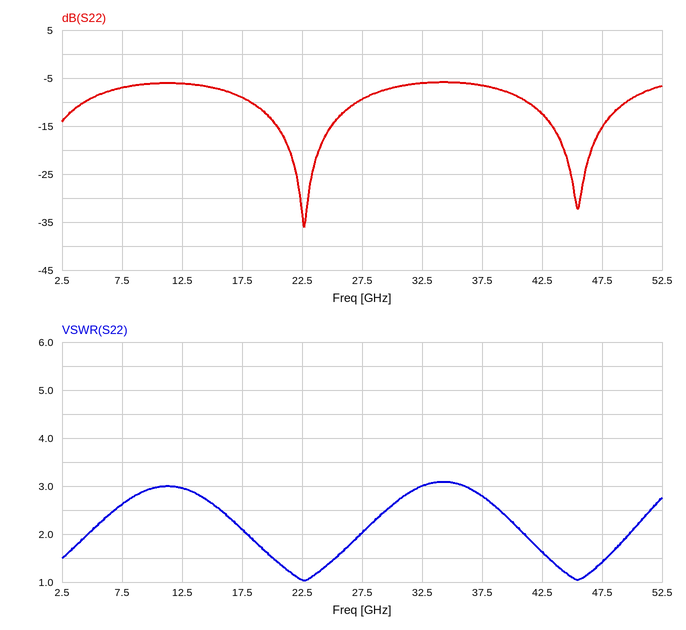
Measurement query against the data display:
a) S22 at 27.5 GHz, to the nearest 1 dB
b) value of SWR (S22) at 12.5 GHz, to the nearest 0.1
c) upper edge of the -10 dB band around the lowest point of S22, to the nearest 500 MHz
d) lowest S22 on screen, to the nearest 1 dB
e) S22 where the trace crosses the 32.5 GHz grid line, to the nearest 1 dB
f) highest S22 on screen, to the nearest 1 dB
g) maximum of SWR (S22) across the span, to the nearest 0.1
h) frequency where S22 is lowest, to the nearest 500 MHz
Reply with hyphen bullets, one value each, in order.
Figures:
- -9 dB
- 3.0
- 27.0 GHz
- -36 dB
- -6 dB
- -6 dB
- 3.1
- 22.5 GHz
